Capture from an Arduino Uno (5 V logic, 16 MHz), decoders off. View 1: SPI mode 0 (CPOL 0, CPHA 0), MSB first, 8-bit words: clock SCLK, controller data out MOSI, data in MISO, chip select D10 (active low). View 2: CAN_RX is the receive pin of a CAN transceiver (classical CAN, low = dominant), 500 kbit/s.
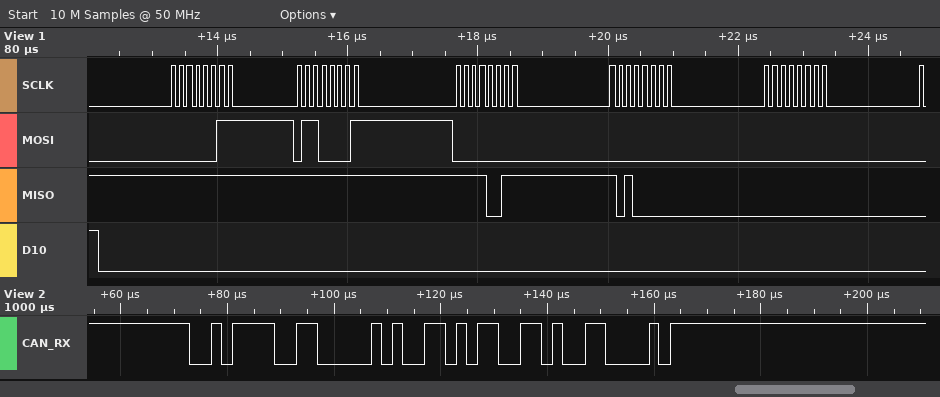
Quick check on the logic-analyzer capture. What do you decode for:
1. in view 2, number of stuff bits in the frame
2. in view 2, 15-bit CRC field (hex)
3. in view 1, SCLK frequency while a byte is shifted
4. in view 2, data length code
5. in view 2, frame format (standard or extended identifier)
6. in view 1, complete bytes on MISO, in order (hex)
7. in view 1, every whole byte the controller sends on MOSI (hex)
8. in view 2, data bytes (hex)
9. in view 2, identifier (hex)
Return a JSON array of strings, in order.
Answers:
["1", "0x4D30", "8 MHz", "1", "standard", "FF FF F3 A0 00", "03 61 00 00 00", "35", "0x2F3"]
